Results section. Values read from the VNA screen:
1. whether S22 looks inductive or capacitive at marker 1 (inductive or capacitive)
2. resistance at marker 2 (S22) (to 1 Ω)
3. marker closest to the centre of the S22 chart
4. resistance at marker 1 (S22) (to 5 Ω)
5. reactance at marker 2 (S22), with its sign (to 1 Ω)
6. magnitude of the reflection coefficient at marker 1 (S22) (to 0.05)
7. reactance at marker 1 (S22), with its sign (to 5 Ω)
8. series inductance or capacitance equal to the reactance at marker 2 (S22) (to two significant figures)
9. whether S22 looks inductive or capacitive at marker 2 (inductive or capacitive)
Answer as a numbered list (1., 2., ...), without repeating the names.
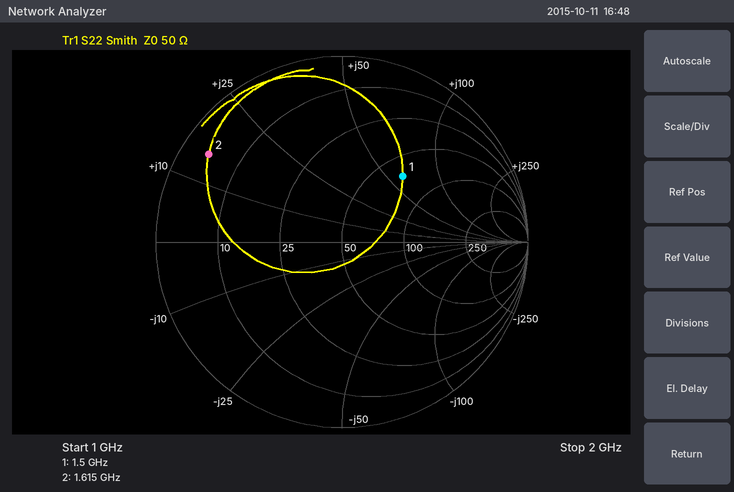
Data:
1. inductive
2. 4 Ω
3. marker 1
4. 65 Ω
5. +15 Ω
6. 0.50
7. +60 Ω
8. 1.5 nH
9. inductive
